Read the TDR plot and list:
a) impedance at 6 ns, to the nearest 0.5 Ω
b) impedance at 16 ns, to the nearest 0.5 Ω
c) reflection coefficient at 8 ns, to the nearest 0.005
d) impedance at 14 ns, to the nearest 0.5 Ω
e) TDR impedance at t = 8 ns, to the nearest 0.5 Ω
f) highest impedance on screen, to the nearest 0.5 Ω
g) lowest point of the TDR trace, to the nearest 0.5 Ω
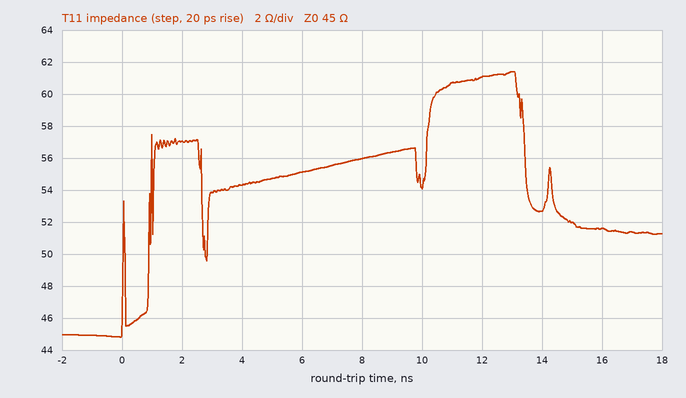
55.0 Ω
51.5 Ω
+0.110
52.5 Ω
56.0 Ω
61.5 Ω
45.0 Ω
